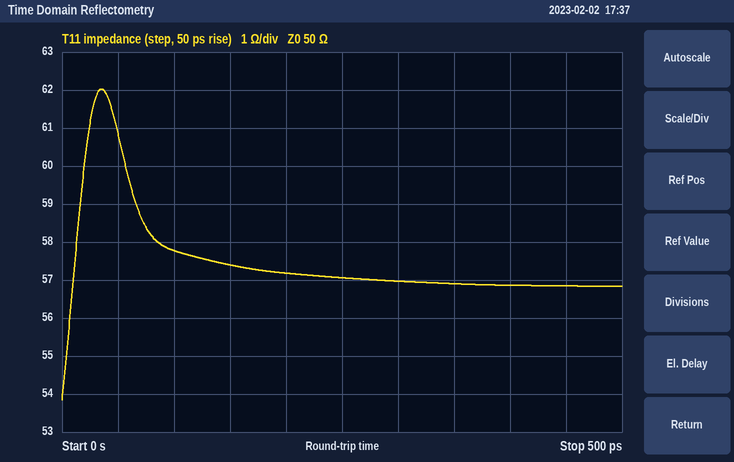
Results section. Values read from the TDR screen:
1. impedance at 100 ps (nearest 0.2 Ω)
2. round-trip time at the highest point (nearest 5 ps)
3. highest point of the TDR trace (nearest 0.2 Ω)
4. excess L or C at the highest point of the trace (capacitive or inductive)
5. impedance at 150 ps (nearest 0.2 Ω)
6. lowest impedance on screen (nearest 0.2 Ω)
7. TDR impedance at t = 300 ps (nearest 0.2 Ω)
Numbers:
57.8 Ω
35 ps
62.0 Ω
inductive
57.4 Ω
53.8 Ω
57.0 Ω
